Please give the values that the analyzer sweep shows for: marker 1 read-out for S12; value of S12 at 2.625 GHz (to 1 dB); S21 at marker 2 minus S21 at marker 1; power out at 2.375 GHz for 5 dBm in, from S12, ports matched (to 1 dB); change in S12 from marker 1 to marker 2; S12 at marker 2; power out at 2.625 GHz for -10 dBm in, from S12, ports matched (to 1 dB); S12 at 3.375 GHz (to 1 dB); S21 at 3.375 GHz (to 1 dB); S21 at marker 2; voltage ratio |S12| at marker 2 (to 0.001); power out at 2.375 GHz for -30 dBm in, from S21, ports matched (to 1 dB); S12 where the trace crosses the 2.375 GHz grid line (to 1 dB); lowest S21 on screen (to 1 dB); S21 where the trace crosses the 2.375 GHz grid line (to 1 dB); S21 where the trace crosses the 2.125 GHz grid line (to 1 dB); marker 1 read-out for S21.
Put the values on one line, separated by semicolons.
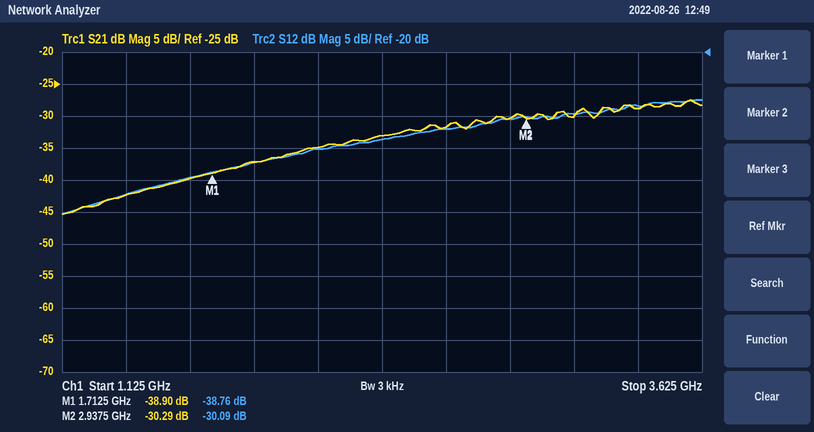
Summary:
-38.76 dB; -32 dB; 8.61 dB; -29 dBm; 8.67 dB; -30.09 dB; -42 dBm; -28 dB; -29 dB; -30.29 dB; 0.031; -63 dBm; -34 dB; -45 dB; -33 dB; -35 dB; -38.90 dB
